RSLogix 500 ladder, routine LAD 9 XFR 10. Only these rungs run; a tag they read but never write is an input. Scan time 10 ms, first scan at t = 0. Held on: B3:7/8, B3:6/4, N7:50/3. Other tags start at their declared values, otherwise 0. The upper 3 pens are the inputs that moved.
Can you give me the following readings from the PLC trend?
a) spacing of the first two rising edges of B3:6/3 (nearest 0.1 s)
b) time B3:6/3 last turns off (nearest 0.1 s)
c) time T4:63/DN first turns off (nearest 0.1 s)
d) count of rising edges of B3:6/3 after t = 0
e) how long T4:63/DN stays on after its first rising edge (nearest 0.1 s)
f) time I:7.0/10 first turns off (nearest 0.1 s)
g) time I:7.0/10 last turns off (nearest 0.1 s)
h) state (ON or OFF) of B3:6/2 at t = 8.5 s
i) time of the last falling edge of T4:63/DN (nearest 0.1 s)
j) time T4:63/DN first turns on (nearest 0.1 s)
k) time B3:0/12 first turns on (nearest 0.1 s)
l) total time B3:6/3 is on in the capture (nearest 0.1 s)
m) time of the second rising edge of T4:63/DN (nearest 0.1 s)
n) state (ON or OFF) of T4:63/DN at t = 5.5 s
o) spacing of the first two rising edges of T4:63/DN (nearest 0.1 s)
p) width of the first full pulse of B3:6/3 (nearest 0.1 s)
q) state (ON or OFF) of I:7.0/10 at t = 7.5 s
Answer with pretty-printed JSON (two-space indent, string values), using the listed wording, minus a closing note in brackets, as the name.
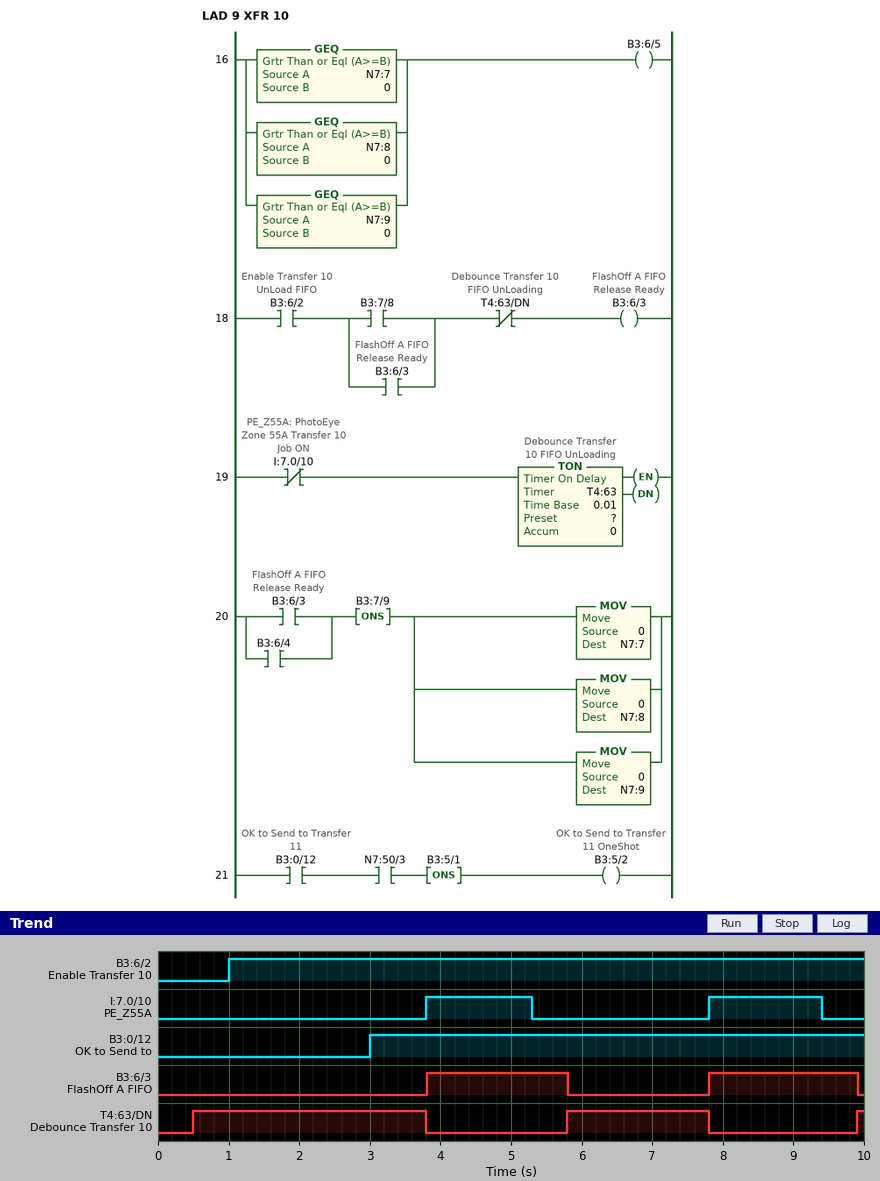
{
  "spacing of the first two rising edges of B3:6/3": "4.0 s",
  "time B3:6/3 last turns off": "9.9 s",
  "time T4:63/DN first turns off": "3.8 s",
  "count of rising edges of B3:6/3 after t = 0": "2",
  "how long T4:63/DN stays on after its first rising edge": "3.3 s",
  "time I:7.0/10 first turns off": "5.3 s",
  "time I:7.0/10 last turns off": "9.4 s",
  "state (ON or OFF) of B3:6/2 at t = 8.5 s": "ON",
  "time of the last falling edge of T4:63/DN": "7.8 s",
  "time T4:63/DN first turns on": "0.5 s",
  "time B3:0/12 first turns on": "3.0 s",
  "total time B3:6/3 is on in the capture": "4.1 s",
  "time of the second rising edge of T4:63/DN": "5.8 s",
  "state (ON or OFF) of T4:63/DN at t = 5.5 s": "OFF",
  "spacing of the first two rising edges of T4:63/DN": "5.3 s",
  "width of the first full pulse of B3:6/3": "2.0 s",
  "state (ON or OFF) of I:7.0/10 at t = 7.5 s": "OFF"
}
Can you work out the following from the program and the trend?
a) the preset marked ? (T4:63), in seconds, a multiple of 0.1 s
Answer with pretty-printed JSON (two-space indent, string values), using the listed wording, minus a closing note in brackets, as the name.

{
  "the preset marked ? (T4:63), in seconds, a multiple of 0.1 s": "0.5 s"
}
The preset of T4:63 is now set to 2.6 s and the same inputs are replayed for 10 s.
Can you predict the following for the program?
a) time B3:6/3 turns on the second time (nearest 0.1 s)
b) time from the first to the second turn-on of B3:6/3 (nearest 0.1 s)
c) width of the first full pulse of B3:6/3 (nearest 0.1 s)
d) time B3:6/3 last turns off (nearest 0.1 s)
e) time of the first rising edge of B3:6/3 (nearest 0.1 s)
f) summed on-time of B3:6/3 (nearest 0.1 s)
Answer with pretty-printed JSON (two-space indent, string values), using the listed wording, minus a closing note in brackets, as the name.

{
  "time B3:6/3 turns on the second time": "3.8 s",
  "time from the first to the second turn-on of B3:6/3": "2.8 s",
  "width of the first full pulse of B3:6/3": "1.6 s",
  "time B3:6/3 last turns off": "2.6 s",
  "time of the first rising edge of B3:6/3": "1.0 s",
  "summed on-time of B3:6/3": "7.8 s"
}
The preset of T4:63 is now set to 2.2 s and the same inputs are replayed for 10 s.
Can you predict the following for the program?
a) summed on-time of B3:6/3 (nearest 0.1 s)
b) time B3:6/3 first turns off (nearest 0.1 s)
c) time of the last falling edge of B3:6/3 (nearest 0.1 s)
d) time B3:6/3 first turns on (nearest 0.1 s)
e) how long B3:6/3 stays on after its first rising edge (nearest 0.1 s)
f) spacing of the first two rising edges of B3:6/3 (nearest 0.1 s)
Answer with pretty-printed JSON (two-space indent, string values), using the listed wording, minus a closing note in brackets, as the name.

{
  "summed on-time of B3:6/3": "7.1 s",
  "time B3:6/3 first turns off": "2.2 s",
  "time of the last falling edge of B3:6/3": "7.5 s",
  "time B3:6/3 first turns on": "1.0 s",
  "how long B3:6/3 stays on after its first rising edge": "1.2 s",
  "spacing of the first two rising edges of B3:6/3": "2.8 s"
}
